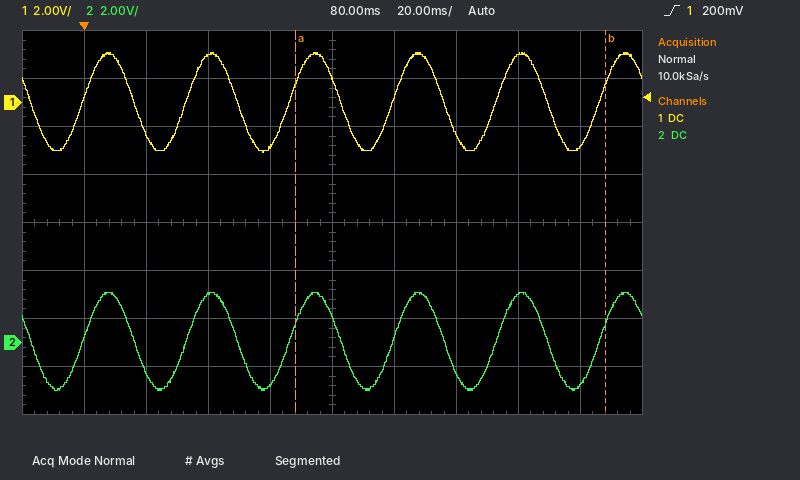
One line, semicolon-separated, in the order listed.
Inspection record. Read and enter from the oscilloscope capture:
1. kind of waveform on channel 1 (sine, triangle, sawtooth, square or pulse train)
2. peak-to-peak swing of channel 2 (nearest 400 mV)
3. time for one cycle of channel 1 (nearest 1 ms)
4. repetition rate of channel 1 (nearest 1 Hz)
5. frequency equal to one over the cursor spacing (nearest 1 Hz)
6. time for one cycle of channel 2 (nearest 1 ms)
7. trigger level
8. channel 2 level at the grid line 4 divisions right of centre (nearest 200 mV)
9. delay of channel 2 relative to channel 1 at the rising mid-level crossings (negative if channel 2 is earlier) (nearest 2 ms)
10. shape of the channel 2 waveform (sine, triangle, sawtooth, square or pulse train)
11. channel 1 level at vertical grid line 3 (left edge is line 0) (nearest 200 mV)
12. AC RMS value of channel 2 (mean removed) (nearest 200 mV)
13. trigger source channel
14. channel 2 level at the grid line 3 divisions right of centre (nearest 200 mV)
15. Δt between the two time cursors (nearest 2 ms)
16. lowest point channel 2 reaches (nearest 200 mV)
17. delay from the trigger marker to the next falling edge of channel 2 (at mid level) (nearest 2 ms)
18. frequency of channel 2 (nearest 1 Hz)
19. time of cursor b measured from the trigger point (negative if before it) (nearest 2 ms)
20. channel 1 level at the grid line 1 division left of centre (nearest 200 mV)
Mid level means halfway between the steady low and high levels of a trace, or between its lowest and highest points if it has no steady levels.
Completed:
sine; 4.0 V; 33 ms; 30 Hz; 10 Hz; 33 ms; 200 mV; -1.8 V; 0 ms; sine; 2.0 V; 1.4 V; channel 1; 2.0 V; 100 ms; -2.0 V; 16 ms; 30 Hz; +168 ms; -1.8 V
